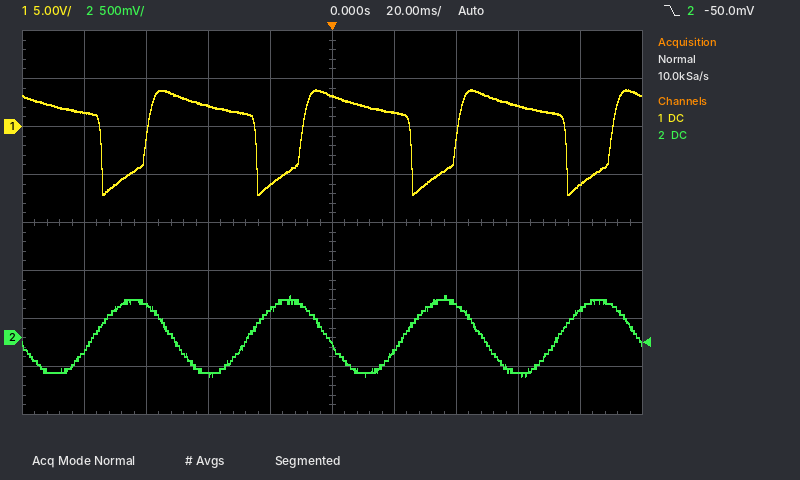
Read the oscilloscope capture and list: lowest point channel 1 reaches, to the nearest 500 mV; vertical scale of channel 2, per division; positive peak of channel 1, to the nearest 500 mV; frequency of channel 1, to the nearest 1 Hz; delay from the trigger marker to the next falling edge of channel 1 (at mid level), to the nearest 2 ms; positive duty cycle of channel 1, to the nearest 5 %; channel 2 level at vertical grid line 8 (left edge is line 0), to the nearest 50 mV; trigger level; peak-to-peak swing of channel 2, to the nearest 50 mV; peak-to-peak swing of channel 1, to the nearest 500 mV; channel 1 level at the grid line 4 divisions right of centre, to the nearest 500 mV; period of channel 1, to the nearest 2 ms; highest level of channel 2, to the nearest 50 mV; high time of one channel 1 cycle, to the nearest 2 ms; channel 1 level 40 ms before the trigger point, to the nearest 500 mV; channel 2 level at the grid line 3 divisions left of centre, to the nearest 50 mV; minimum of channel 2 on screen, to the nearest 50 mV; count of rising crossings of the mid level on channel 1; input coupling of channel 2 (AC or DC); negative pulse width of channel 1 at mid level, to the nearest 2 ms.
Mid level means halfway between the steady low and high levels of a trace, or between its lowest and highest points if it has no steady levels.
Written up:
-7.0 V
500 mV
4.0 V
20 Hz
26 ms
70 %
-350 mV
-50.0 mV
850 mV
11.0 V
-6.0 V
50 ms
450 mV
36 ms
2.0 V
350 mV
-400 mV
4
DC
14 ms
